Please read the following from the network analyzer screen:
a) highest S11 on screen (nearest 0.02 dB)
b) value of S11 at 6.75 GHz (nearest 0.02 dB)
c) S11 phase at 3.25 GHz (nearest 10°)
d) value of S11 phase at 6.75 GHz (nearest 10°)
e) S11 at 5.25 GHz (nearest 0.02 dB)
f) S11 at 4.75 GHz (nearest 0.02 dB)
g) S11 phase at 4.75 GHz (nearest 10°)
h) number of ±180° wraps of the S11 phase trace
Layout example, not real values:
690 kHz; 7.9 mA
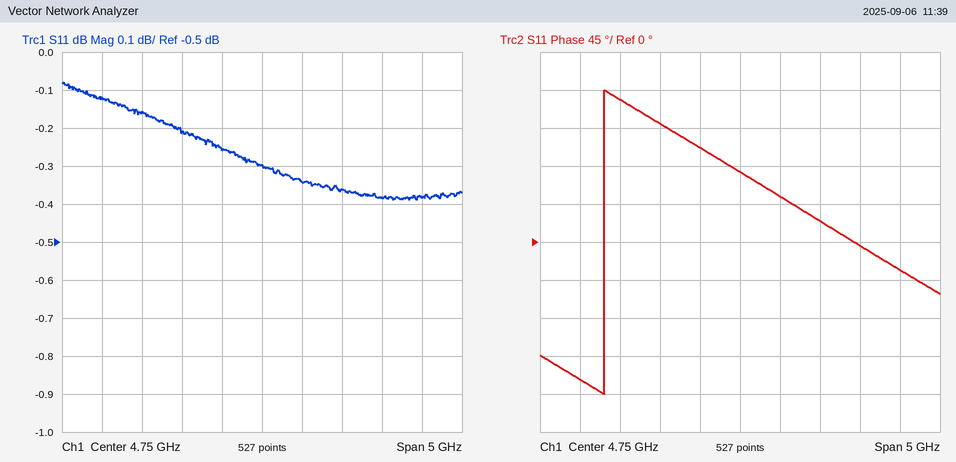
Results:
-0.08 dB; -0.38 dB; 170°; -30°; -0.34 dB; -0.30 dB; 80°; 1
